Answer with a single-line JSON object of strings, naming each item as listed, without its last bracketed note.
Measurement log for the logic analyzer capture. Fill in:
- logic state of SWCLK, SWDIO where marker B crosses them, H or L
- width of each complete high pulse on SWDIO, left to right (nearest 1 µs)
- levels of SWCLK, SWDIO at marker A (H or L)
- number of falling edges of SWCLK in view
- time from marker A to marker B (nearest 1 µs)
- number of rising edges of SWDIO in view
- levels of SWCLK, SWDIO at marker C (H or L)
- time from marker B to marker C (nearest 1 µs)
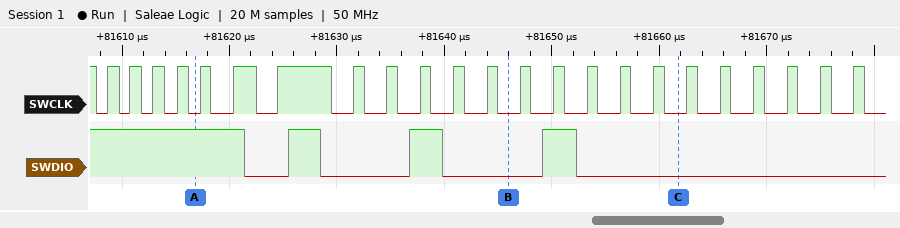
{"logic state of SWCLK, SWDIO where marker B crosses them, H or L": "SWCLK=L, SWDIO=L", "width of each complete high pulse on SWDIO, left to right": "3 µs, 3 µs, 3 µs", "levels of SWCLK, SWDIO at marker A": "SWCLK=L, SWDIO=H", "number of falling edges of SWCLK in view": "24", "time from marker A to marker B": "29 µs", "number of rising edges of SWDIO in view": "3", "levels of SWCLK, SWDIO at marker C": "SWCLK=L, SWDIO=L", "time from marker B to marker C": "16 µs"}
